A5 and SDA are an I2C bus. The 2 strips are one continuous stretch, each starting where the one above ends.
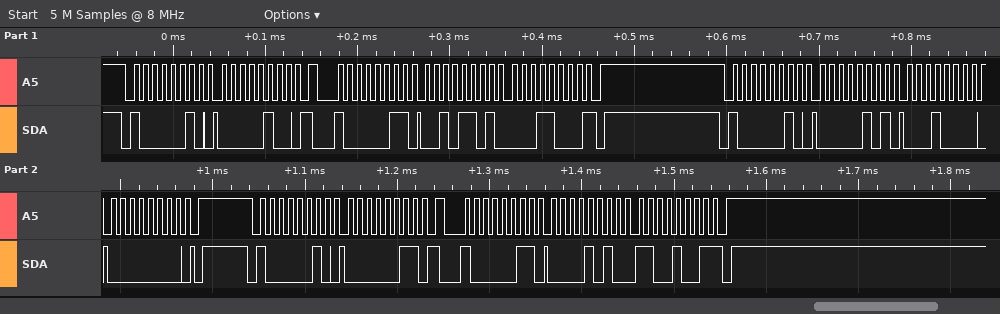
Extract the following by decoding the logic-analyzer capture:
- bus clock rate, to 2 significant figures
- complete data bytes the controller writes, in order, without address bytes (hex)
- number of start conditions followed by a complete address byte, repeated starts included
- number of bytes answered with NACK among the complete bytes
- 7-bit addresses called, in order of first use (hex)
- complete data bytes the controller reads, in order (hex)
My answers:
100 kHz
04 05 10 00 03
5
2
0x41
2D 18 0A C9
